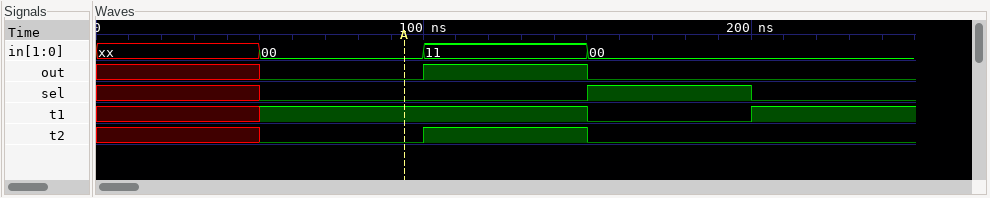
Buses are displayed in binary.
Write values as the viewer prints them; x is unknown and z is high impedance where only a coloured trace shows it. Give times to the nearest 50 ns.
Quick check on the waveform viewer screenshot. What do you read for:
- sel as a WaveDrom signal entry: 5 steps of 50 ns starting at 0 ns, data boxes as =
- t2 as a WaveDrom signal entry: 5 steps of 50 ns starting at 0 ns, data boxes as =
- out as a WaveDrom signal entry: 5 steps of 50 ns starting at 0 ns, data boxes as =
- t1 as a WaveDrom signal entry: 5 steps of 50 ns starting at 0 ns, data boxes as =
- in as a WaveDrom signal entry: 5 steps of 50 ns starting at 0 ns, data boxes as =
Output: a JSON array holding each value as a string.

["{name: 'sel', wave: 'x0.10'}", "{name: 't2', wave: 'x010.'}", "{name: 'out', wave: 'x010.'}", "{name: 't1', wave: 'x1.01'}", "{name: 'in', wave: 'x===.', data: '00 11 00'}"]
